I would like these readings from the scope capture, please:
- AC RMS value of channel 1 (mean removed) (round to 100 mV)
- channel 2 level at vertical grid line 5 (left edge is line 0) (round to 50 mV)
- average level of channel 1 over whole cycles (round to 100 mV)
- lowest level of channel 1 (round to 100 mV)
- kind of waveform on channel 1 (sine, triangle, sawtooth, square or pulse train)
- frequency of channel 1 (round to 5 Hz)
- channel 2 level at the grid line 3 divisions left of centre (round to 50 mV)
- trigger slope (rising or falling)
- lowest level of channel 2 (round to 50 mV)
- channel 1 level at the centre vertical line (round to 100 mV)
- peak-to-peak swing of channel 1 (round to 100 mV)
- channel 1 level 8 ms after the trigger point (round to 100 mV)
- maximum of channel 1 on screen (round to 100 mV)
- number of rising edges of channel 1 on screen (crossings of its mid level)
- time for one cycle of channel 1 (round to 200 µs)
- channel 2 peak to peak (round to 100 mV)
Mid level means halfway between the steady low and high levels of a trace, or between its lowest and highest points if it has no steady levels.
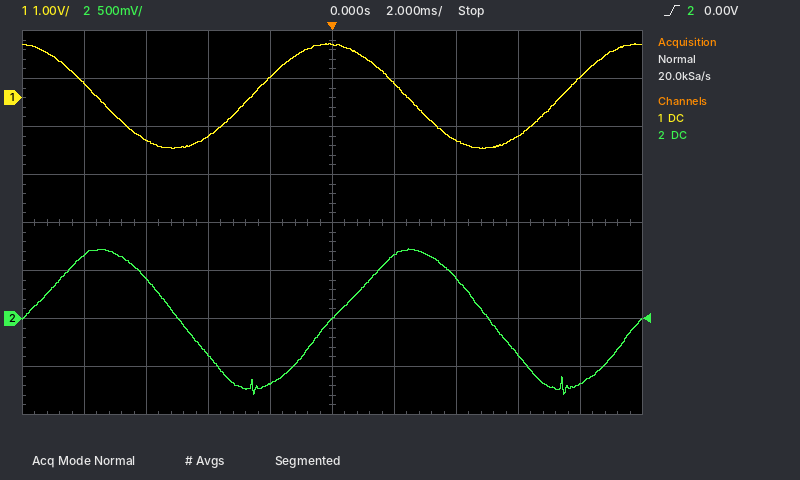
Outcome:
800 mV
0 mV
0.0 V
-1.1 V
sine
100 Hz
400 mV
rising
-800 mV
1.1 V
2.2 V
400 mV
1.1 V
2
10.0 ms
1.50 V
